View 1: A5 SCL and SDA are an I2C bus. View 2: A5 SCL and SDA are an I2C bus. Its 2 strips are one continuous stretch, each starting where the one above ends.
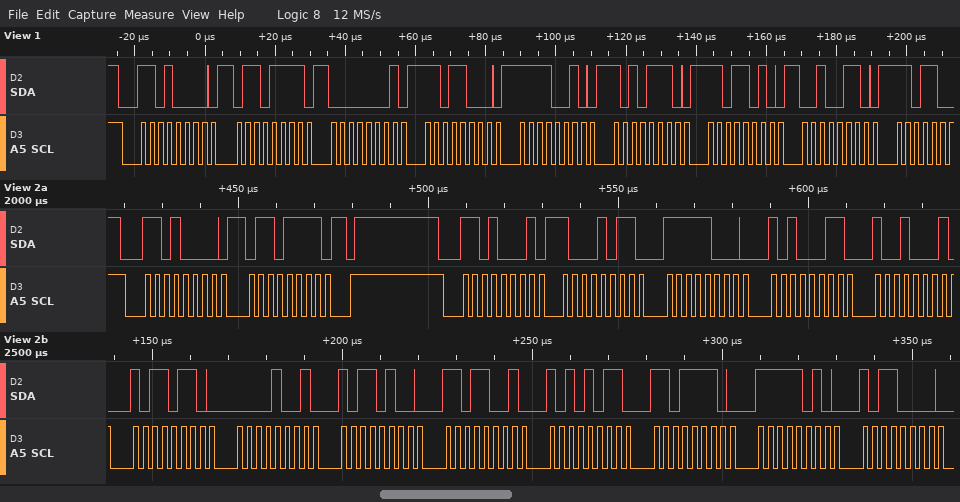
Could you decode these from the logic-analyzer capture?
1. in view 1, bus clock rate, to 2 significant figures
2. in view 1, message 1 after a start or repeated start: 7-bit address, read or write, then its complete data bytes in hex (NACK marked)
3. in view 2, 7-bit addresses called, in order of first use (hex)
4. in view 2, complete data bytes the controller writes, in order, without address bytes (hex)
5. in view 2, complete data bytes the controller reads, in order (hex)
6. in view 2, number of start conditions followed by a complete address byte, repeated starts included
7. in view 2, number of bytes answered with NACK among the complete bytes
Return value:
400 kHz
0x68 write: 6F 01 D8 F2 AE DA 26
0x68
6F
8B F8 A3 91 B6 09 B4 D9 AB DE FA B0
2
0
